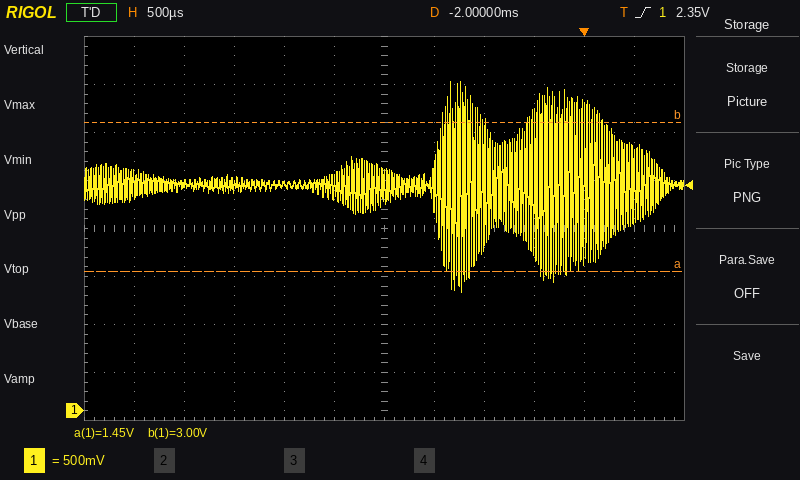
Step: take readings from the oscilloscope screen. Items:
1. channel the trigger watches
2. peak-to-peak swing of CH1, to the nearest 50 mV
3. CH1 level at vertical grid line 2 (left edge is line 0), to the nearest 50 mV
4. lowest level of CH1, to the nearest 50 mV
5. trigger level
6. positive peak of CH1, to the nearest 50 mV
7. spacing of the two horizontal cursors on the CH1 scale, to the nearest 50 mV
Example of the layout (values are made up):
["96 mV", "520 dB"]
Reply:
["CH1", "2.20 V", "2.35 V", "1.25 V", "2.35 V", "3.45 V", "1.55 V"]
